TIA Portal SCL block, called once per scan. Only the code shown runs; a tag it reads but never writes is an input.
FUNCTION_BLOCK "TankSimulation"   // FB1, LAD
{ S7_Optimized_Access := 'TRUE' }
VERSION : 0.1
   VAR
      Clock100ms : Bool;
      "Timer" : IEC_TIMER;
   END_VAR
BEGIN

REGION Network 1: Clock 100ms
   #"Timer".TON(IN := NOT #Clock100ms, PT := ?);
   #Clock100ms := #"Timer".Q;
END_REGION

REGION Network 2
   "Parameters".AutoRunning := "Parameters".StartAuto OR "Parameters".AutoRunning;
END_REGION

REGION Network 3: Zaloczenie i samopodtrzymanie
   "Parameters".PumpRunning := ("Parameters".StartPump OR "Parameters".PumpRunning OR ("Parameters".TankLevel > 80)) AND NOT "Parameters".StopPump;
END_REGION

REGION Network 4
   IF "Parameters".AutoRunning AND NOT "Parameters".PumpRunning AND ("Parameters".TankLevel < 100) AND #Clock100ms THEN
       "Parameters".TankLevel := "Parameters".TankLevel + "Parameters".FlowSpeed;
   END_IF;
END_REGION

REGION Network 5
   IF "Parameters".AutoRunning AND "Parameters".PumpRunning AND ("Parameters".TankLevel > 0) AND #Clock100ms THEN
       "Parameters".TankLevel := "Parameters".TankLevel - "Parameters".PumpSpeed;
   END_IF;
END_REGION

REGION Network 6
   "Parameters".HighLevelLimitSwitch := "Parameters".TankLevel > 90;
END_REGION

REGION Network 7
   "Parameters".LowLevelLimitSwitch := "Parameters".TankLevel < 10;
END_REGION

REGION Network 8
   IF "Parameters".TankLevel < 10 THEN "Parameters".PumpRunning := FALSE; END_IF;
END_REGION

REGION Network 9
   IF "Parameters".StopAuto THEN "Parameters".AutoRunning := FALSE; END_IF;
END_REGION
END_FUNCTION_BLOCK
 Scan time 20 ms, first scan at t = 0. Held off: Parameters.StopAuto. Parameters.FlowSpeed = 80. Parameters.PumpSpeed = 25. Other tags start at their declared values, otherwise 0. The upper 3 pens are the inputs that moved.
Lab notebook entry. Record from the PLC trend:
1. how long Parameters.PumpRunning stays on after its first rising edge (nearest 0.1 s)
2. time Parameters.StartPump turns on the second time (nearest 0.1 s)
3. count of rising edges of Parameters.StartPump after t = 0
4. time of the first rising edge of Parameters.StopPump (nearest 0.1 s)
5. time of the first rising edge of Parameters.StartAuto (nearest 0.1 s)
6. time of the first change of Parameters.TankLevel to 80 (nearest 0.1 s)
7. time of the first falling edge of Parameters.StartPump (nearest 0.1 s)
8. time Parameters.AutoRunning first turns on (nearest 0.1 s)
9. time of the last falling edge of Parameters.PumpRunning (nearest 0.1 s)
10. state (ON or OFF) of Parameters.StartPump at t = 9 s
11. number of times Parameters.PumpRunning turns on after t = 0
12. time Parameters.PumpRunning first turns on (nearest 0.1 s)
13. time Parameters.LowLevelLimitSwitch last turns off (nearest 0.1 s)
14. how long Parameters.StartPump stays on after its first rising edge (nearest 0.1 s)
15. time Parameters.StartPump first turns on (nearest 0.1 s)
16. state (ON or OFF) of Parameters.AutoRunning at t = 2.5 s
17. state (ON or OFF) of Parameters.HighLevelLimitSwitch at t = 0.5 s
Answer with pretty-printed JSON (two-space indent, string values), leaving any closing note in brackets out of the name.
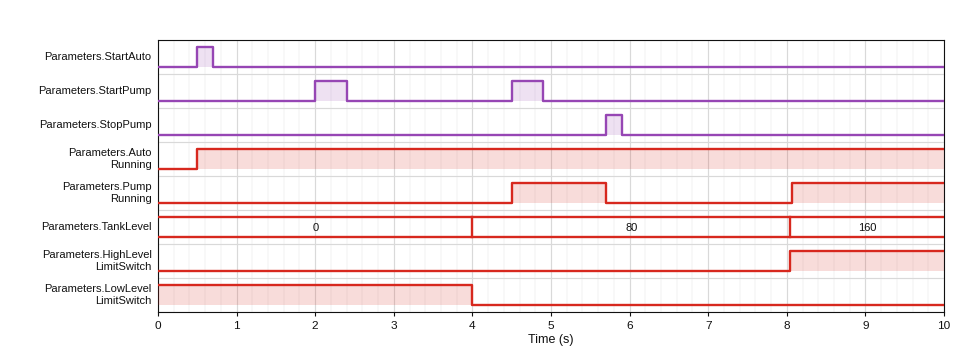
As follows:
{
  "how long Parameters.PumpRunning stays on after its first rising edge": "1.2 s",
  "time Parameters.StartPump turns on the second time": "4.5 s",
  "count of rising edges of Parameters.StartPump after t = 0": "2",
  "time of the first rising edge of Parameters.StopPump": "5.7 s",
  "time of the first rising edge of Parameters.StartAuto": "0.5 s",
  "time of the first change of Parameters.TankLevel to 80": "4.0 s",
  "time of the first falling edge of Parameters.StartPump": "2.4 s",
  "time Parameters.AutoRunning first turns on": "0.5 s",
  "time of the last falling edge of Parameters.PumpRunning": "5.7 s",
  "state (ON or OFF) of Parameters.StartPump at t = 9 s": "OFF",
  "number of times Parameters.PumpRunning turns on after t = 0": "2",
  "time Parameters.PumpRunning first turns on": "4.5 s",
  "time Parameters.LowLevelLimitSwitch last turns off": "4.0 s",
  "how long Parameters.StartPump stays on after its first rising edge": "0.4 s",
  "time Parameters.StartPump first turns on": "2.0 s",
  "state (ON or OFF) of Parameters.AutoRunning at t = 2.5 s": "ON",
  "state (ON or OFF) of Parameters.HighLevelLimitSwitch at t = 0.5 s": "OFF"
}
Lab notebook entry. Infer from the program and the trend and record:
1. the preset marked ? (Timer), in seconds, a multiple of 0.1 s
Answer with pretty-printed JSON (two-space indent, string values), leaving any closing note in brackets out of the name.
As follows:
{
  "the preset marked ? (Timer), in seconds, a multiple of 0.1 s": "4.0 s"
}
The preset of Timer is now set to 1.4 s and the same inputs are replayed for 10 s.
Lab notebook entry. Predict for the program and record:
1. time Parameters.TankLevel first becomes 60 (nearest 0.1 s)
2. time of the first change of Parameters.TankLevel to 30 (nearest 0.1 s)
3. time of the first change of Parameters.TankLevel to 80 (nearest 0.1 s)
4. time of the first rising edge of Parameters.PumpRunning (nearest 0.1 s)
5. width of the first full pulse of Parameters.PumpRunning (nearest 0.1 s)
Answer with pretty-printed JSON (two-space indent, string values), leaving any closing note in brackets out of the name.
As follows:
{
  "time Parameters.TankLevel first becomes 60": "8.6 s",
  "time of the first change of Parameters.TankLevel to 30": "4.3 s",
  "time of the first change of Parameters.TankLevel to 80": "1.4 s",
  "time of the first rising edge of Parameters.PumpRunning": "2.0 s",
  "width of the first full pulse of Parameters.PumpRunning": "3.7 s"
}
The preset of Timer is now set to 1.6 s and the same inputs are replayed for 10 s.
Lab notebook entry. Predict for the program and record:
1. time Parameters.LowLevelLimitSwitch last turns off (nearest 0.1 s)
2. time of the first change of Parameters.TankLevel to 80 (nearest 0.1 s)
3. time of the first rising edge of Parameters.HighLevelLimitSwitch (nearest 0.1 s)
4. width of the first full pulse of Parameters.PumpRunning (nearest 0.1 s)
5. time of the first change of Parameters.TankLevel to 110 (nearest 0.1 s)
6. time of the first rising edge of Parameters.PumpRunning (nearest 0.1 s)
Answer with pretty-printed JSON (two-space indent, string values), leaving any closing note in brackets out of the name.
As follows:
{
  "time Parameters.LowLevelLimitSwitch last turns off": "1.6 s",
  "time of the first change of Parameters.TankLevel to 80": "1.6 s",
  "time of the first rising edge of Parameters.HighLevelLimitSwitch": "6.5 s",
  "width of the first full pulse of Parameters.PumpRunning": "3.7 s",
  "time of the first change of Parameters.TankLevel to 110": "6.5 s",
  "time of the first rising edge of Parameters.PumpRunning": "2.0 s"
}
